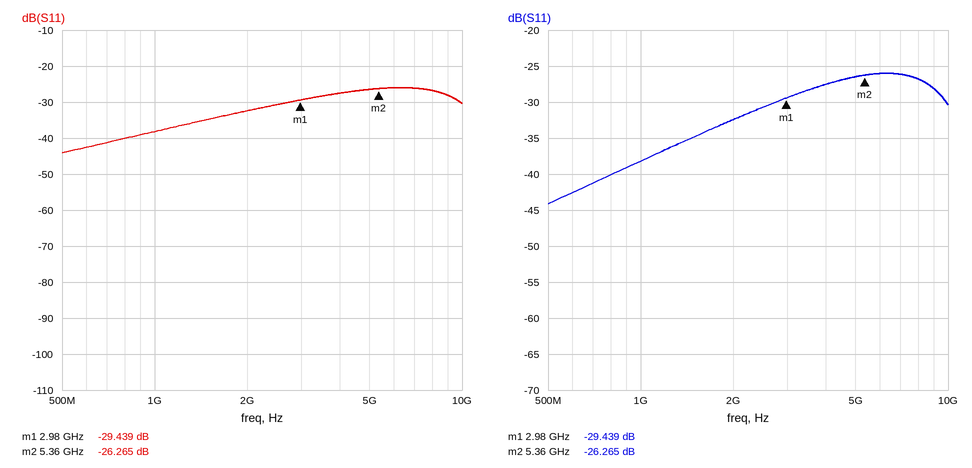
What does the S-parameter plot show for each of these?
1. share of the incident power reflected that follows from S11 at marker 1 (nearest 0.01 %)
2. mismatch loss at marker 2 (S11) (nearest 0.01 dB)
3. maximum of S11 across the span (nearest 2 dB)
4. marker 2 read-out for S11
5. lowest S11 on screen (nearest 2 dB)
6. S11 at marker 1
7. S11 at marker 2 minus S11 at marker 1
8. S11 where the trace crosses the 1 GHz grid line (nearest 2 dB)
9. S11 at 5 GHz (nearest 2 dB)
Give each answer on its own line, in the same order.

0.11 %
0.01 dB
-26 dB
-26.265 dB
-44 dB
-29.439 dB
3.174 dB
-38 dB
-26 dB
